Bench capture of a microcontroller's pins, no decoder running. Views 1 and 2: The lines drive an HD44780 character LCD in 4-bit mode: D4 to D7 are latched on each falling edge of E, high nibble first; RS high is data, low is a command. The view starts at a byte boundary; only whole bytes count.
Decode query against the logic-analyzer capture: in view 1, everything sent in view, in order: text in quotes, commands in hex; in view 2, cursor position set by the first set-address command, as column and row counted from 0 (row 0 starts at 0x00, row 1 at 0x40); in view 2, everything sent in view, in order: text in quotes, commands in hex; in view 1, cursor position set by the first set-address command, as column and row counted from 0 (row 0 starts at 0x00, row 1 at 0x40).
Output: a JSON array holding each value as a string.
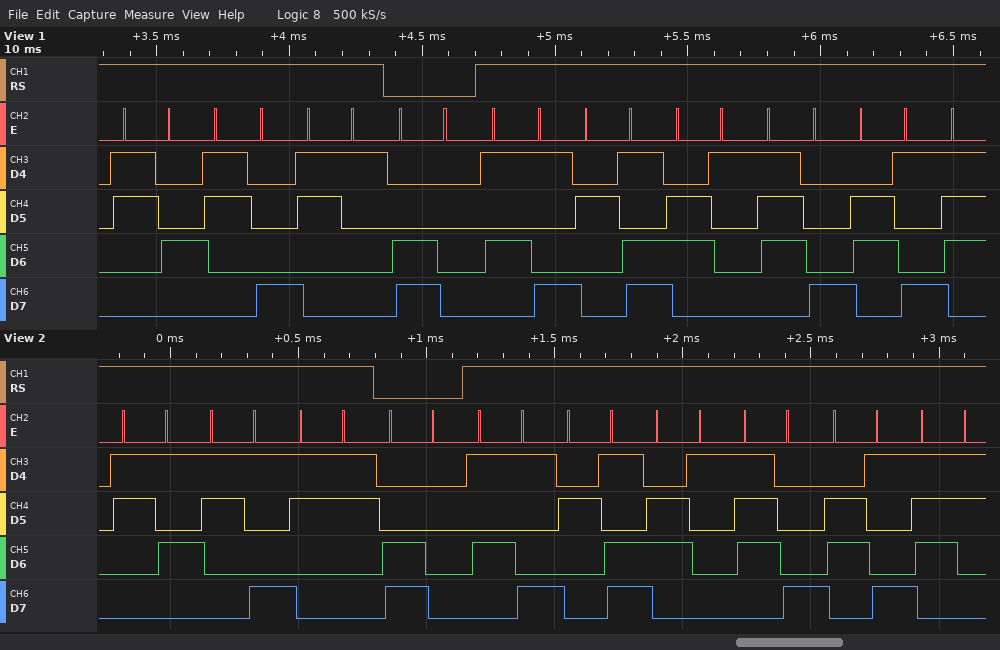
["\"481\" 0xC0 \"Y-axi\"", "column 0, row 1", "\"593\" 0xC0 \"Y-axis\"", "column 0, row 1"]
